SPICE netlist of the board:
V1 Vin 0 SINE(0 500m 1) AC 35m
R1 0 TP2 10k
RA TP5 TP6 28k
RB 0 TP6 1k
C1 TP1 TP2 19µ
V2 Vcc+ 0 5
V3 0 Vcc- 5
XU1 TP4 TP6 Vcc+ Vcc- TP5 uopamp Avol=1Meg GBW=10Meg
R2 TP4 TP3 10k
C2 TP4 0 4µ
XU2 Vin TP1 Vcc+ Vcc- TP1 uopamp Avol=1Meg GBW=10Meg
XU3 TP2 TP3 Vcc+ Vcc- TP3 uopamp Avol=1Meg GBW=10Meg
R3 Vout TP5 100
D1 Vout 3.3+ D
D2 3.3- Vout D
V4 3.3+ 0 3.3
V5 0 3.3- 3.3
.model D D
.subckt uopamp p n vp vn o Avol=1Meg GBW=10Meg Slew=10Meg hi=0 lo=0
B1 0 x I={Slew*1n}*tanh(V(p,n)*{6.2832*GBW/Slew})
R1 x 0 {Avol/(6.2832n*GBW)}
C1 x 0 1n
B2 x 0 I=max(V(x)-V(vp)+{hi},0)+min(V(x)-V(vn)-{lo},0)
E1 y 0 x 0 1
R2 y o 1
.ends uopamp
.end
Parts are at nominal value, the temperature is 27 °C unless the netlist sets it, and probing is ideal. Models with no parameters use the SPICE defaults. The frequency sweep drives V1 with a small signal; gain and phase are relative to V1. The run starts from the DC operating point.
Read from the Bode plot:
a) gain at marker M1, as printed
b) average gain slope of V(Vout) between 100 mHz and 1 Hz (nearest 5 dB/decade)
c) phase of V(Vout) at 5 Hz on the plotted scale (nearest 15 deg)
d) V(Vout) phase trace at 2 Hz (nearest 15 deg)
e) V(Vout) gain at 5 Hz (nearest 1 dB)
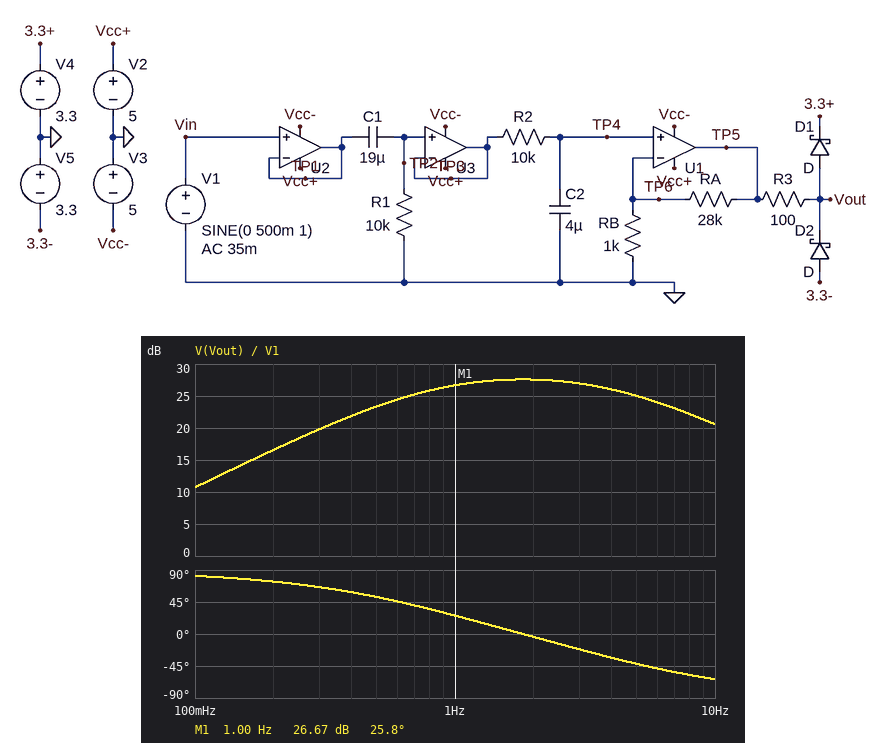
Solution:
26.67 dB
15 dB/decade
-45 deg
0 deg
25 dB
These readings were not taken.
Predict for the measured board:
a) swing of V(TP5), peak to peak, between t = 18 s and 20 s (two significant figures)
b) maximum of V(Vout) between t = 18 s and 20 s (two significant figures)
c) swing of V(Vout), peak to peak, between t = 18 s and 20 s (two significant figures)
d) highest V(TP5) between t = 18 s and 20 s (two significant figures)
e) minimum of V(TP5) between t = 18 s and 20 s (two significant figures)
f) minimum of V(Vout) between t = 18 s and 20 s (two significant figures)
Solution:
10 V
4.0 V
8.0 V
5.0 V
-5.0 V
-4.0 V
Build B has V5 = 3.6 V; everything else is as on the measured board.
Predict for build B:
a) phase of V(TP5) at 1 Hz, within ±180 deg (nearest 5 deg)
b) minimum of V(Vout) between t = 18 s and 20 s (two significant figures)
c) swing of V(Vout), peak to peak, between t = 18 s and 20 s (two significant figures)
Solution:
25 deg
-4.3 V
8.3 V
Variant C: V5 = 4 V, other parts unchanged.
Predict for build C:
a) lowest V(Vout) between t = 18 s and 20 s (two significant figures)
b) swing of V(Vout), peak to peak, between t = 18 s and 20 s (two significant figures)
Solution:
-4.7 V
8.7 V
